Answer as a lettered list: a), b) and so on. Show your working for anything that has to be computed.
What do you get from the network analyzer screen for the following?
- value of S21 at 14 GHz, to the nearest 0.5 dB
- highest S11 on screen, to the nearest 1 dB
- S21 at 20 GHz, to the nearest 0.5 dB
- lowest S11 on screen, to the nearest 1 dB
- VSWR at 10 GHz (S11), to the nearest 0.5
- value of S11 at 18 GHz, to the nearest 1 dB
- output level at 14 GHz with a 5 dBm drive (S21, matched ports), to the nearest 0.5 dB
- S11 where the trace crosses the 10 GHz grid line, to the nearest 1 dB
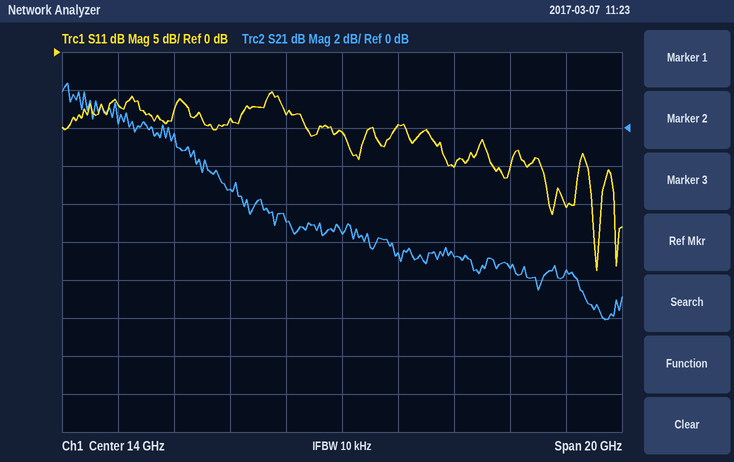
a) -5.5 dB
b) -5 dB
c) -7.5 dB
d) -29 dB
e) |Γ| = 10^(-9/20) = 0.3548; VSWR = (1 + 0.3548)/(1 − 0.3548) ≈ 2.10, so 2.0 to the nearest 0.5
f) -15 dB
g) 5 dBm + (-5.5 dB) = -0.5 dBm
h) -9 dB
